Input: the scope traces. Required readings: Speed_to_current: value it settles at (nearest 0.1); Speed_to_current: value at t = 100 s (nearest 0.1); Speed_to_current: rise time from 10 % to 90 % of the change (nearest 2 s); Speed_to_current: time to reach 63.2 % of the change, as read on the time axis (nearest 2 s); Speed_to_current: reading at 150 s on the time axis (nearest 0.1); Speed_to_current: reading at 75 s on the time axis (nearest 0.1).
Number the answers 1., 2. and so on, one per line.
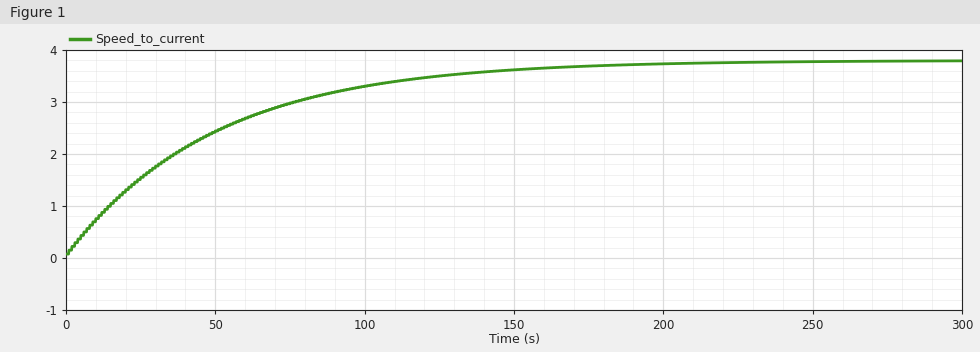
1. 3.8
2. 3.3
3. 108 s
4. 50 s
5. 3.6
6. 3.0
